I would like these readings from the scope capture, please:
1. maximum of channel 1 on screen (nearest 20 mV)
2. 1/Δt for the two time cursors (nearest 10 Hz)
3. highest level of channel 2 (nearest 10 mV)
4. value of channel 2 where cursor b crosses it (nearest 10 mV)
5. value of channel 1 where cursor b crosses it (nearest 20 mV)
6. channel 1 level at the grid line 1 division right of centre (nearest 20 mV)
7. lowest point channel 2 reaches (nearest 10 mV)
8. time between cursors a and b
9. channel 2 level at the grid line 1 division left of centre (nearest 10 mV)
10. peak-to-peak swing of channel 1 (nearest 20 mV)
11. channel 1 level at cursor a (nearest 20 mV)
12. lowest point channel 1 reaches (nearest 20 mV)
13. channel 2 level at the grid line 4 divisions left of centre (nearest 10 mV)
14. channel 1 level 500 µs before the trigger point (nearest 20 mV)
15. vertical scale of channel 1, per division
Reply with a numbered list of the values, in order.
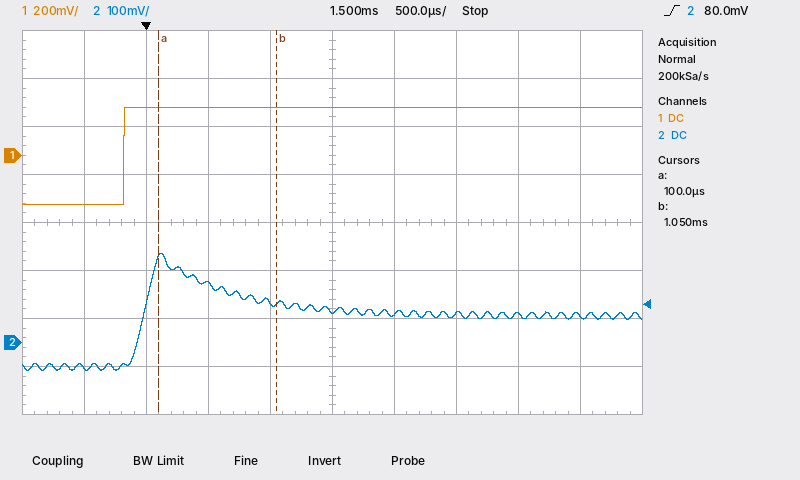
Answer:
1. 200 mV
2. 1.05 kHz
3. 190 mV
4. 80 mV
5. 200 mV
6. 200 mV
7. -60 mV
8. 950 µs
9. 80 mV
10. 400 mV
11. 200 mV
12. -200 mV
13. -50 mV
14. -200 mV
15. 200 mV
